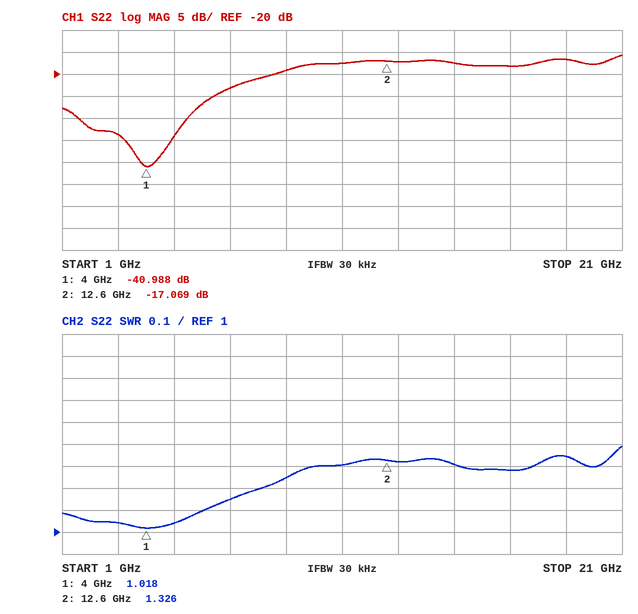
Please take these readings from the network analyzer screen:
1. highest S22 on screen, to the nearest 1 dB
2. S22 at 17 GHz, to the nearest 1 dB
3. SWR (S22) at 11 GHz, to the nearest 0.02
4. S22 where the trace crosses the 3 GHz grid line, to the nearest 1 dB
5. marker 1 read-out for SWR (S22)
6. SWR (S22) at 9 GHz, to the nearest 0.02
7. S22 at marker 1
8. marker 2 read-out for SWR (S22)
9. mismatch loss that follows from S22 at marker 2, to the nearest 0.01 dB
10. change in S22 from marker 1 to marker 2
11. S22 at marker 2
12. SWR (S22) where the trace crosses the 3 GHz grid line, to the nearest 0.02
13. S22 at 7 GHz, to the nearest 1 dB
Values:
-16 dB
-18 dB
1.30
-34 dB
1.018
1.24
-40.988 dB
1.326
0.09 dB
23.919 dB
-17.069 dB
1.04
-23 dB
